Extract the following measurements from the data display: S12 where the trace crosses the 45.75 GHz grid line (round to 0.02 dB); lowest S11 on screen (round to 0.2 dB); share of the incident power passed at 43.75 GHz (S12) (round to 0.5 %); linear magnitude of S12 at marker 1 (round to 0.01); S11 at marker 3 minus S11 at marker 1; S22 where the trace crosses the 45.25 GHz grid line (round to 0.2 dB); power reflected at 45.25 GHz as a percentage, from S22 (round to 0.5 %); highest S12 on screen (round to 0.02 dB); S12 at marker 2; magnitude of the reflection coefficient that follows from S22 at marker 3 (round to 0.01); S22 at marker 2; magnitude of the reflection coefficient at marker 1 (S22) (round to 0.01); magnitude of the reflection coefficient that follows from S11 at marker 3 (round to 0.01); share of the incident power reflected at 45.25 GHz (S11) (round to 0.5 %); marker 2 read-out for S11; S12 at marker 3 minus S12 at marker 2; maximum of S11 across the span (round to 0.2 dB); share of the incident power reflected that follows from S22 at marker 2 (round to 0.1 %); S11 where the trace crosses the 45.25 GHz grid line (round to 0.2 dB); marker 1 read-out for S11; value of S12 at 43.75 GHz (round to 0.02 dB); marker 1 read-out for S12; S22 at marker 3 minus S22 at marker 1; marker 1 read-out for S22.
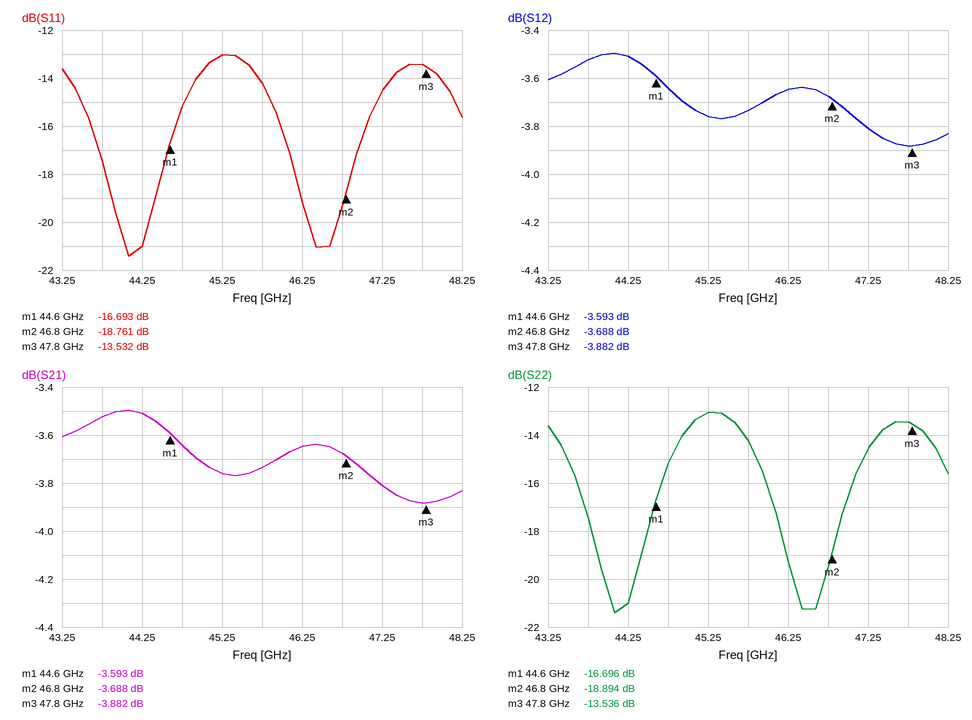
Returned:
-3.74 dB
-21.4 dB
44.5 %
0.66
3.161 dB
-13.0 dB
5.0 %
-3.50 dB
-3.688 dB
0.21
-18.894 dB
0.15
0.21
5.0 %
-18.761 dB
-0.194 dB
-13.0 dB
1.3 %
-13.0 dB
-16.693 dB
-3.52 dB
-3.593 dB
3.160 dB
-16.696 dB
